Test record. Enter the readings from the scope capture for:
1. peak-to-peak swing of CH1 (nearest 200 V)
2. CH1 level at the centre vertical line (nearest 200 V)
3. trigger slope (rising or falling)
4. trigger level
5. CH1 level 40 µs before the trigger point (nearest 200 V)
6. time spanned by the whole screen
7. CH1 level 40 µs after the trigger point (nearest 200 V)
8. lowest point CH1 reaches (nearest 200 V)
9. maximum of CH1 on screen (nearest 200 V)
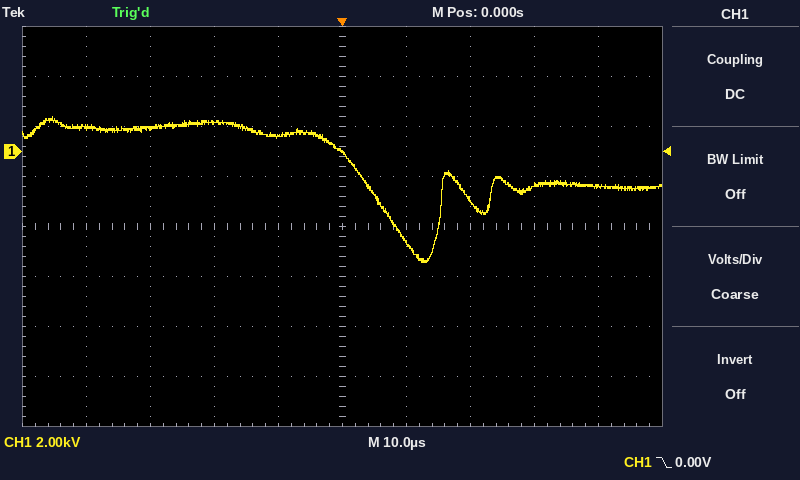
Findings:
5.8 kV
0.0 kV
falling
0.00 V
1.0 kV
100 µs
-1.4 kV
-4.4 kV
1.4 kV
